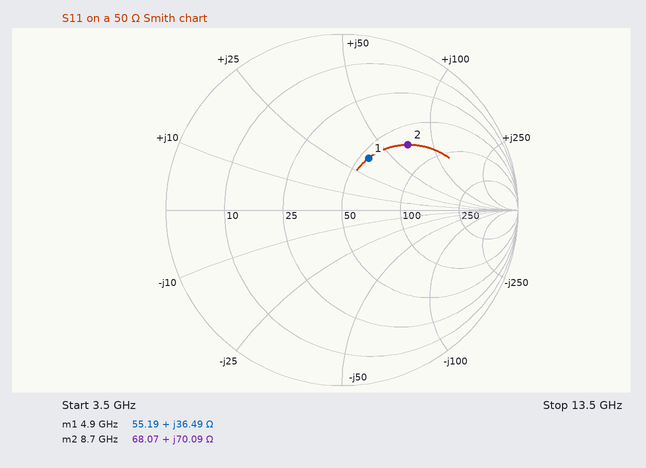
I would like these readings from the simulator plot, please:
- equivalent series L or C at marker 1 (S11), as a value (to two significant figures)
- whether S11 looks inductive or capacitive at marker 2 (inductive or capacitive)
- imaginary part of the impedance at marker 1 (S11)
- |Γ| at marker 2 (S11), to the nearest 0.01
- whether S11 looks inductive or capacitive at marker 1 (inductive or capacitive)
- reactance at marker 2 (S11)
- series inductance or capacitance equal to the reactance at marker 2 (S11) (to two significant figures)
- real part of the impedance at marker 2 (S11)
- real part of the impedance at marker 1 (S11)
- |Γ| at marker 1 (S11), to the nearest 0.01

1.2 nH
inductive
+36.49 Ω
0.53
inductive
+70.09 Ω
1.3 nH
68.07 Ω
55.19 Ω
0.33
